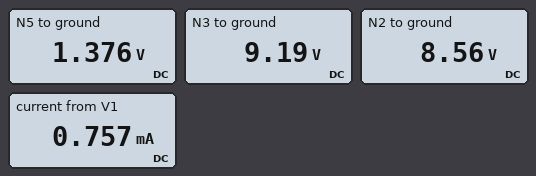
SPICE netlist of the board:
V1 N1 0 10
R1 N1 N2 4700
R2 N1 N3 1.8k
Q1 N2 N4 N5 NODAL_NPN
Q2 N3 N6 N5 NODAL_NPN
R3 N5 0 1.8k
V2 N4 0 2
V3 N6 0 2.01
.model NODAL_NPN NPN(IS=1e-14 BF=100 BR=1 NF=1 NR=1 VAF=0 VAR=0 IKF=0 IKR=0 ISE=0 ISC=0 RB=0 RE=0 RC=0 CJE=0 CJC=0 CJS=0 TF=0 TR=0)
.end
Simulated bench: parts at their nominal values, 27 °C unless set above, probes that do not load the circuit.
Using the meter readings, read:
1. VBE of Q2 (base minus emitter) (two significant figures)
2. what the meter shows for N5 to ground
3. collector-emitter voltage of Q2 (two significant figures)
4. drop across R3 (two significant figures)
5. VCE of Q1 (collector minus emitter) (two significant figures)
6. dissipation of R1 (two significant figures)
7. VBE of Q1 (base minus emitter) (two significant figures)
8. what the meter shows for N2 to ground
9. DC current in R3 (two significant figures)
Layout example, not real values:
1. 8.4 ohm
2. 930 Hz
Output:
1. 630 mV
2. 1.376 V
3. 7.8 V
4. 1.4 V
5. 7.2 V
6. 440 µW
7. 620 mV
8. 8.56 V
9. 760 µA
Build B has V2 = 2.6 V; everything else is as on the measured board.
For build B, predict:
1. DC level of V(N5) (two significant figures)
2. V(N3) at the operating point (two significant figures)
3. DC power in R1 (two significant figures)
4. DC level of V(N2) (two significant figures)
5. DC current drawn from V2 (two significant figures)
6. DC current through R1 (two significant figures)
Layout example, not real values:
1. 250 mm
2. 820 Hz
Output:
1. 1.9 V
2. 10 V
3. 5.4 mW
4. 5.0 V
5. 11 µA
6. 1.1 mA
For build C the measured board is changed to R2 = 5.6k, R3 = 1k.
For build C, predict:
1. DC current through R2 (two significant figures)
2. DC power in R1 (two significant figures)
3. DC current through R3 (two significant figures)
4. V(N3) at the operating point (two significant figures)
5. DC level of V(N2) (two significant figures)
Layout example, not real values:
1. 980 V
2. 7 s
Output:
1. 800 µA
2. 1.4 mW
3. 1.4 mA
4. 5.5 V
5. 7.4 V
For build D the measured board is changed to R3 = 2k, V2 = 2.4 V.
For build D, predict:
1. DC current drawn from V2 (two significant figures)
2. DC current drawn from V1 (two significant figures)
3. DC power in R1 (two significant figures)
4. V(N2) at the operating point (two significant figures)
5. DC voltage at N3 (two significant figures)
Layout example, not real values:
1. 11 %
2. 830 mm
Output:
1. 8.7 µA
2. 870 µA
3. 3.5 mW
4. 5.9 V
5. 10 V
